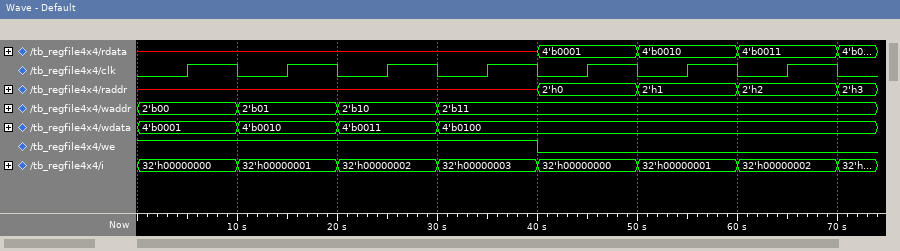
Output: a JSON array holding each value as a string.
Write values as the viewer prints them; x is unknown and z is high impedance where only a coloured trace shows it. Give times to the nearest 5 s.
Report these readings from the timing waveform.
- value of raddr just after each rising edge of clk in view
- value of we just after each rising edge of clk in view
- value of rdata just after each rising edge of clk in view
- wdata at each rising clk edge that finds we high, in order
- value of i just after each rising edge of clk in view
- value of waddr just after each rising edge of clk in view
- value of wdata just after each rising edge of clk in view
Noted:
["x, x, x, x, 2'h0, 2'h1, 2'h2", "1 1 1 1 0 0 0", "x, x, x, x, 4'b0001, 4'b0010, 4'b0011", "4'b0001, 4'b0010, 4'b0011, 4'b0100", "32'h00000000, 32'h00000001, 32'h00000002, 32'h00000003, 32'h00000000, 32'h00000001, 32'h00000002", "2'b00, 2'b01, 2'b10, 2'b11, 2'b11, 2'b11, 2'b11", "4'b0001, 4'b0010, 4'b0011, 4'b0100, 4'b0100, 4'b0100, 4'b0100"]
